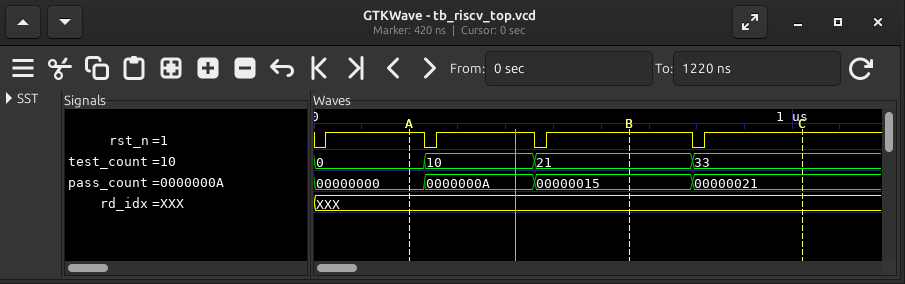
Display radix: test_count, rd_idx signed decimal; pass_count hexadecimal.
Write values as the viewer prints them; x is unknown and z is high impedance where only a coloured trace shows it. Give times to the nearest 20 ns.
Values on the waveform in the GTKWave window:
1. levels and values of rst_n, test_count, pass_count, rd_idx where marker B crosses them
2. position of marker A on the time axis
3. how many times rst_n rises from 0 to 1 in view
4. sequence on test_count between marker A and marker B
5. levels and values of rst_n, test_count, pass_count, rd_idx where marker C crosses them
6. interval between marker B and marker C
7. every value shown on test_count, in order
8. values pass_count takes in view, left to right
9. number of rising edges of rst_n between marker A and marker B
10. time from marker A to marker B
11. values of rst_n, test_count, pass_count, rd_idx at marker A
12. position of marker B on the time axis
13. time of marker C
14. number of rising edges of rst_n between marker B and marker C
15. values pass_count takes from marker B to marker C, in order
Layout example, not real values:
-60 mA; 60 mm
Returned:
rst_n=1, test_count=21, pass_count=00000015, rd_idx=XXX; 200 ns; 4; 0, 10, 21; rst_n=1, test_count=33, pass_count=00000021, rd_idx=XXX; 360 ns; 0, 10, 21, 33; 00000000, 0000000A, 00000015, 00000021; 2; 460 ns; rst_n=1, test_count=0, pass_count=00000000, rd_idx=XXX; 660 ns; 1020 ns; 1; 00000015, 00000021
